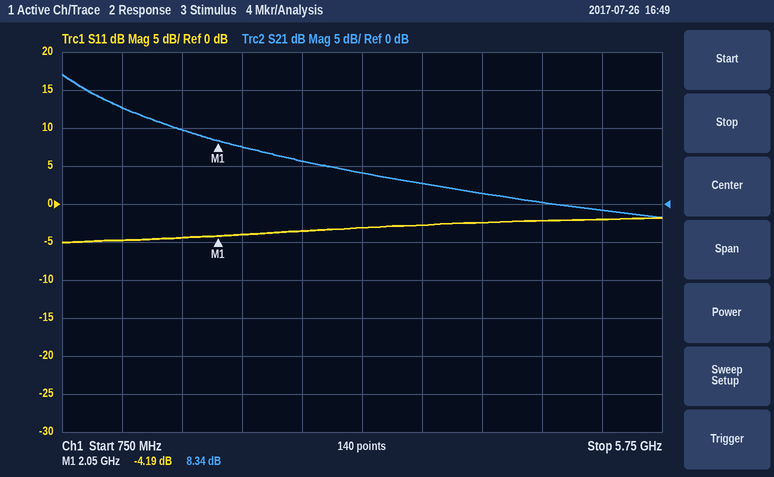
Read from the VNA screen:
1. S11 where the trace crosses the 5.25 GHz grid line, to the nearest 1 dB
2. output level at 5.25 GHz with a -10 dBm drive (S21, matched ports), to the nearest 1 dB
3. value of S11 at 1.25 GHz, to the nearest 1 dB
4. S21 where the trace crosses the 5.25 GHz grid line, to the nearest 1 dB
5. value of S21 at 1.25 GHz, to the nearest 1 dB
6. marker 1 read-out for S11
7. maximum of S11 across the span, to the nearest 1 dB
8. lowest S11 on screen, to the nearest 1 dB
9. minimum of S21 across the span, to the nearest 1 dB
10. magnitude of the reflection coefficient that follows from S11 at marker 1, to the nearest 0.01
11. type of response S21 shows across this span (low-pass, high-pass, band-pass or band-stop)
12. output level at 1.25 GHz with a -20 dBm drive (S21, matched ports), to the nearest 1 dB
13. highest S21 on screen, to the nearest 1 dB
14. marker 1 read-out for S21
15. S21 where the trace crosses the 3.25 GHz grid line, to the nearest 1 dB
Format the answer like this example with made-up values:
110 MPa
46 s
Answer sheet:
-2 dB
-11 dBm
-5 dB
-1 dB
13 dB
-4.19 dB
-2 dB
-5 dB
-2 dB
0.62
low-pass
-7 dBm
17 dB
8.34 dB
4 dB
